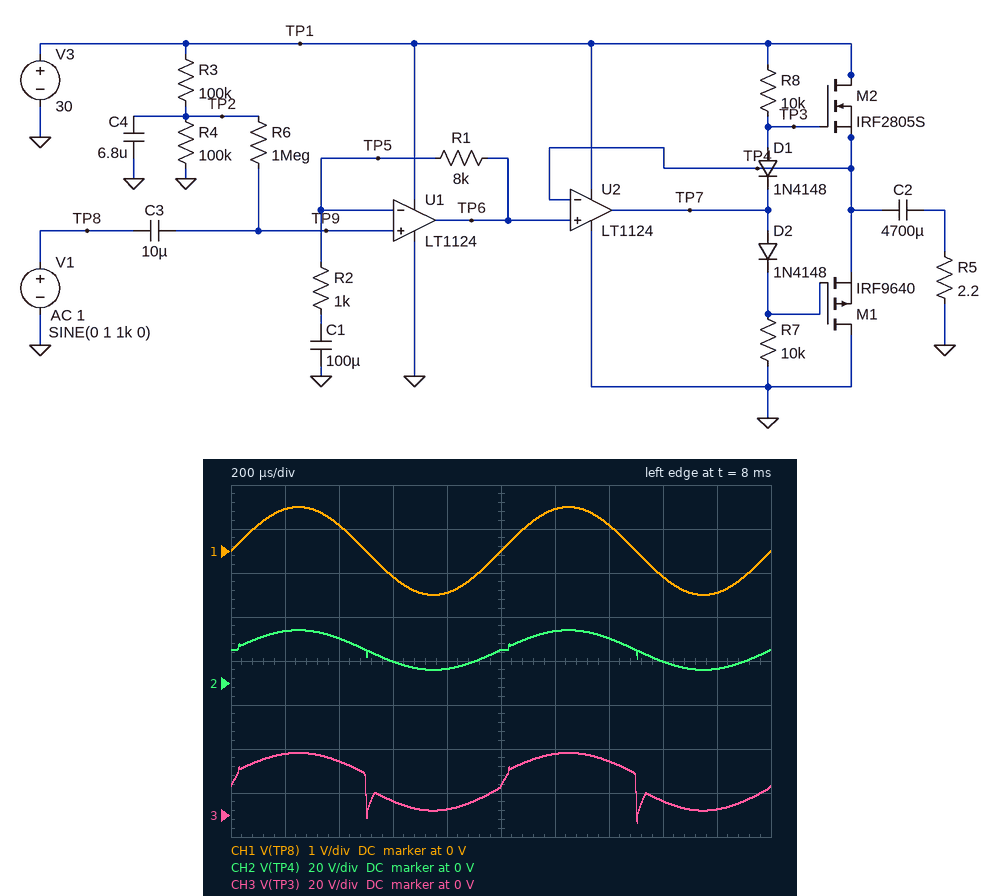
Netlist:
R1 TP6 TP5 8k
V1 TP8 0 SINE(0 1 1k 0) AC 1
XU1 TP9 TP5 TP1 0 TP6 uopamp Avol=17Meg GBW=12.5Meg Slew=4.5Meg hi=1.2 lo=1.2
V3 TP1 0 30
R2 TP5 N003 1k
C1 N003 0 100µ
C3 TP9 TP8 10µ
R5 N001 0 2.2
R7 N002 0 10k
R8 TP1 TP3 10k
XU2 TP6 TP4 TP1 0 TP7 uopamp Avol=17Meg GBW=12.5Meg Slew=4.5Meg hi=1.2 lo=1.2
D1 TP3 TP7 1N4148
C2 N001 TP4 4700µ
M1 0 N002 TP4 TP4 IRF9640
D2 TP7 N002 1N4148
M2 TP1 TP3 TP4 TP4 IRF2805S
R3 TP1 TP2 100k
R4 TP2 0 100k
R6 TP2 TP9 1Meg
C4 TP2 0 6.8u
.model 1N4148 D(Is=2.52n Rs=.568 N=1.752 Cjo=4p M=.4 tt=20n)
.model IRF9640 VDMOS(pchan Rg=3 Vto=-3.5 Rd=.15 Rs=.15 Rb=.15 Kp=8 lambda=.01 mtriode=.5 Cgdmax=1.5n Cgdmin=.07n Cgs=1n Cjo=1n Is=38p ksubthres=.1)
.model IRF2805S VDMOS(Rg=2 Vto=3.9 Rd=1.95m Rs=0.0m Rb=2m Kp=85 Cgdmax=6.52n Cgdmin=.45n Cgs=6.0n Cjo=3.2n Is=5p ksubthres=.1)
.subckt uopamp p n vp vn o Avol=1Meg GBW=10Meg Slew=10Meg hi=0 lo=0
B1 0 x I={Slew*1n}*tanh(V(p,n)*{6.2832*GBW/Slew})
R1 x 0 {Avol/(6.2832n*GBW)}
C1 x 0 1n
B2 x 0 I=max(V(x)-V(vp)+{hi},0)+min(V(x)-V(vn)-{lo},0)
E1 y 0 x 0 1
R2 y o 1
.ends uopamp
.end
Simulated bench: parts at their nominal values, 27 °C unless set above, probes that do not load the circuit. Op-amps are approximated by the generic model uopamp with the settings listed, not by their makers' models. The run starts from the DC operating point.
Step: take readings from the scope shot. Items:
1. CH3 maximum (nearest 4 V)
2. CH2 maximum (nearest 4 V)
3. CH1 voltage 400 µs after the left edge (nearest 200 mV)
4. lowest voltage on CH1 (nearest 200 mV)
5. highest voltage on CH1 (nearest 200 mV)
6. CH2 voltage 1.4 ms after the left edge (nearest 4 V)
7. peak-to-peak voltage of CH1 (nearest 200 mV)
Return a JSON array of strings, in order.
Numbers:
["28 V", "24 V", "600 mV", "-1.0 V", "1.0 V", "20 V", "2.0 V"]
